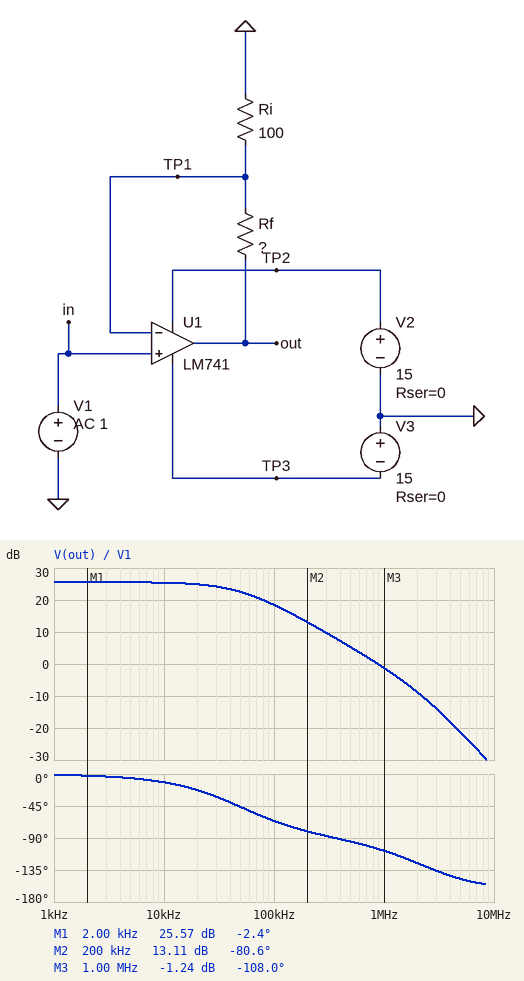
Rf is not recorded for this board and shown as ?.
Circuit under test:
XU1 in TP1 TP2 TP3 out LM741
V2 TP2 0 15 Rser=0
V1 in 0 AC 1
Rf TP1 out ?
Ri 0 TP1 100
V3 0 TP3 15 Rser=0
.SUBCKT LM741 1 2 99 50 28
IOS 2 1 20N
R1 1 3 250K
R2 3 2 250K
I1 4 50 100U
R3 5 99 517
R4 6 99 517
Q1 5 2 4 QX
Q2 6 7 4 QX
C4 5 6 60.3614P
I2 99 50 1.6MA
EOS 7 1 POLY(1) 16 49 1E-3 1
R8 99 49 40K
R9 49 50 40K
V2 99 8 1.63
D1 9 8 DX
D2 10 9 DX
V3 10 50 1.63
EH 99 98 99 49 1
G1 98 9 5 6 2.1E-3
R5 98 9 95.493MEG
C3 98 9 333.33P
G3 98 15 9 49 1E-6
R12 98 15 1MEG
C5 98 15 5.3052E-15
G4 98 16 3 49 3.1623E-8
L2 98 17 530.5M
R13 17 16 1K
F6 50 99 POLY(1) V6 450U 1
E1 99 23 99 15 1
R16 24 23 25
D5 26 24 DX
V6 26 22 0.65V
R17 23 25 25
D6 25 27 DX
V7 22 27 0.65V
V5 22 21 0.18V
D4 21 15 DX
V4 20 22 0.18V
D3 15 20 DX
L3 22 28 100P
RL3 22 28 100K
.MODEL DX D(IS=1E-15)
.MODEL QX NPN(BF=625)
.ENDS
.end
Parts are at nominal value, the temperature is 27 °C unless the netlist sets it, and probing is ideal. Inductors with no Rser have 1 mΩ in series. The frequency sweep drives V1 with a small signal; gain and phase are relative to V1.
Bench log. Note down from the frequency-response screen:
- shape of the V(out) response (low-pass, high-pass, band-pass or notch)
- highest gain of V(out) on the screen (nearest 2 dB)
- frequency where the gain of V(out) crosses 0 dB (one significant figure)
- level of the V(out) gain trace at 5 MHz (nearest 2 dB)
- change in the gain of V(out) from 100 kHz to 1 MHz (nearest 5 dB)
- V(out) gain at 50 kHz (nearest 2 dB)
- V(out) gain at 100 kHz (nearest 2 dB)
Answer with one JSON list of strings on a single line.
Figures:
["low-pass", "26 dB", "900 kHz", "-22 dB", "-20 dB", "22 dB", "18 dB"]
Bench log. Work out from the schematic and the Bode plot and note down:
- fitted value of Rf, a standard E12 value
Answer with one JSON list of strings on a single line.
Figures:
["1.8 kΩ"]
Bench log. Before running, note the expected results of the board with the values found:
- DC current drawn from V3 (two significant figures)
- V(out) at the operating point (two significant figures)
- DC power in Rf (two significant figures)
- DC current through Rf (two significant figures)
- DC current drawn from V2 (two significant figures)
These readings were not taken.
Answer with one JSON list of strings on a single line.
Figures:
["1.7 mA", "19 mV", "180 nW", "10 µA", "1.7 mA"]
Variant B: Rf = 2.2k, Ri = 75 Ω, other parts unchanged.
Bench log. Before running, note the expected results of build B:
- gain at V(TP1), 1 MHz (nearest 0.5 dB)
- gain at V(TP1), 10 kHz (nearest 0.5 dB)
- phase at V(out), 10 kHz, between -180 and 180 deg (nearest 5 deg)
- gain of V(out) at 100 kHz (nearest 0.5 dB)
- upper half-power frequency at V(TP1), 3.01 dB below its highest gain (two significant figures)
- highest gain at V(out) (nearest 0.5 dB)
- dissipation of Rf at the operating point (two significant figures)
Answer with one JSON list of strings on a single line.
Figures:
["-31.0 dB", "-0.5 dB", "-20 deg", "19.0 dB", "31 kHz", "29.5 dB", "400 nW"]
